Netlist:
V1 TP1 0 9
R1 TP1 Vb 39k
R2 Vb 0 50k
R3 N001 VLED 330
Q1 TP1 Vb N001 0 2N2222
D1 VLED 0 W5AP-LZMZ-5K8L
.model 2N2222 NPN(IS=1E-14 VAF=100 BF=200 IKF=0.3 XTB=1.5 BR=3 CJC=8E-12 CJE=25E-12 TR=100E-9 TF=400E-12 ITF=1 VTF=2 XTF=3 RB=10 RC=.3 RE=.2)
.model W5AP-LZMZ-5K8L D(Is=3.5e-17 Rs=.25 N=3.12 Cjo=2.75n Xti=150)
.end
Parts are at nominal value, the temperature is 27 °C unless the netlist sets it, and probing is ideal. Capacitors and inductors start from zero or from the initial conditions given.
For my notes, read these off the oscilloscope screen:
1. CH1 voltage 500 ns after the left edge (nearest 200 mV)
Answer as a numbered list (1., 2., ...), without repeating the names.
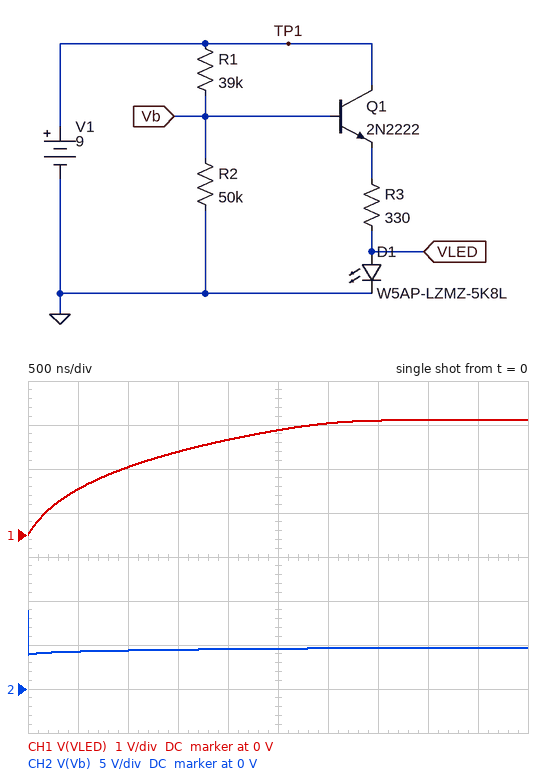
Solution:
1. 1.0 V
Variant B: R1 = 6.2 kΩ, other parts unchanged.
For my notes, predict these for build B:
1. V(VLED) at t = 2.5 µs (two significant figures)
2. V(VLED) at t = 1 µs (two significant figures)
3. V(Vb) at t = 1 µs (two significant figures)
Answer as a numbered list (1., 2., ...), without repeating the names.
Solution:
1. 2.7 V
2. 2.4 V
3. 7.6 V
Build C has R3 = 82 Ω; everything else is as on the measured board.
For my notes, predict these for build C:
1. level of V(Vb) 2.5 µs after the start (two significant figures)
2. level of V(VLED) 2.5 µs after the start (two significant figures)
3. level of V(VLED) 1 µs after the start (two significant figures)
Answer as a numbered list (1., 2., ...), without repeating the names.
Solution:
1. 4.1 V
2. 2.7 V
3. 2.3 V
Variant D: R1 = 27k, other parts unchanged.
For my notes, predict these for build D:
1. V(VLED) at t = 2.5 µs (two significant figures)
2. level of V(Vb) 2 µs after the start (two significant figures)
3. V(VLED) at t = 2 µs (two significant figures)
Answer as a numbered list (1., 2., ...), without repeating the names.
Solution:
1. 2.6 V
2. 5.3 V
3. 2.5 V
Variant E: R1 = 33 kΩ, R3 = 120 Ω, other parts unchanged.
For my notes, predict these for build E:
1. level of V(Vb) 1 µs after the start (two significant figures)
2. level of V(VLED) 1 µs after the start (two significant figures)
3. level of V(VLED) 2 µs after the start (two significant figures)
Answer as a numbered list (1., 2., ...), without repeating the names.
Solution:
1. 4.3 V
2. 2.3 V
3. 2.7 V
